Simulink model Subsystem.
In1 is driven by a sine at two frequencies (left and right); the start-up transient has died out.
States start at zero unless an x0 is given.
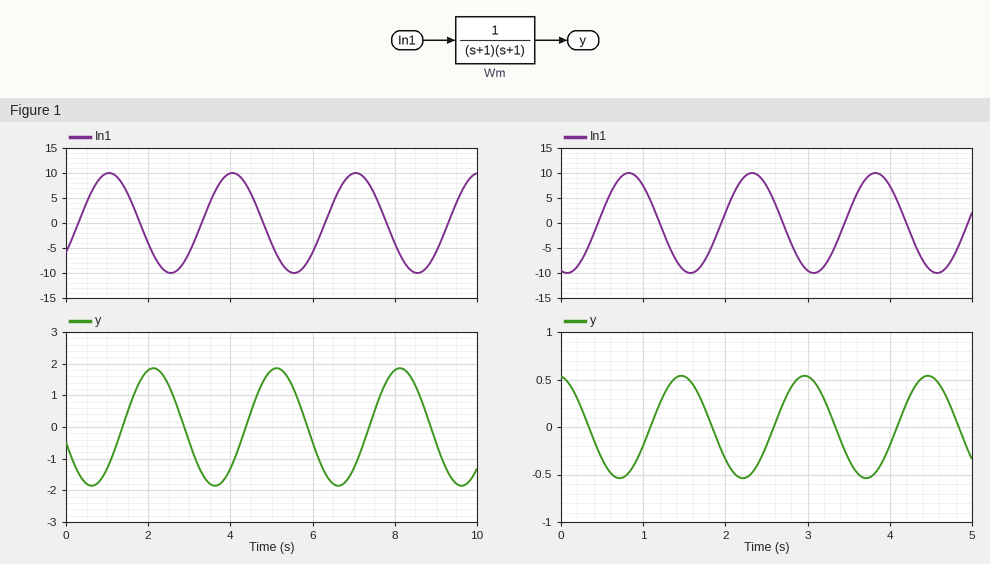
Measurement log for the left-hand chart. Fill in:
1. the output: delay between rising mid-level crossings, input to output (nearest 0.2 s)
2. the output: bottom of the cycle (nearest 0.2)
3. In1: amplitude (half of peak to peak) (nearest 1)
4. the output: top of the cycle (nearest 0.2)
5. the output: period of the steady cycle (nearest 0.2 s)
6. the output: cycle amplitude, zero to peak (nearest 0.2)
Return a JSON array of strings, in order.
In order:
["1.0 s", "-1.8", "10", "1.8", "3.0 s", "1.8"]
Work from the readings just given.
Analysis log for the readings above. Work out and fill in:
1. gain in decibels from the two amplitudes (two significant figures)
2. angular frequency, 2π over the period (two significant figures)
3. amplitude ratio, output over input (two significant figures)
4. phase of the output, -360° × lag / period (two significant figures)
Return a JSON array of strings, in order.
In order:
["-15 dB", "2.1 rad/s", "0.18", "-120°"]
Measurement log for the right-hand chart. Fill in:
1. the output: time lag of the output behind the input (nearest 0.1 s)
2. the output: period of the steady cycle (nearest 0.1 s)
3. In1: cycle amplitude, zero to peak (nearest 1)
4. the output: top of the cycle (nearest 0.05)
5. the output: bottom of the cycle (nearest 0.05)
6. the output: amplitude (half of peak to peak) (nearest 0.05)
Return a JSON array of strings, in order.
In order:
["0.6 s", "1.5 s", "10", "0.55", "-0.55", "0.55"]
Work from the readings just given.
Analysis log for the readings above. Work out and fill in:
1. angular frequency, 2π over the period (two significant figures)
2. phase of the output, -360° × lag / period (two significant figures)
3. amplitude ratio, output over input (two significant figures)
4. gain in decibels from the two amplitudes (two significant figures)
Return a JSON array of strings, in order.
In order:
["4.2 rad/s", "-140°", "0.055", "-25 dB"]
